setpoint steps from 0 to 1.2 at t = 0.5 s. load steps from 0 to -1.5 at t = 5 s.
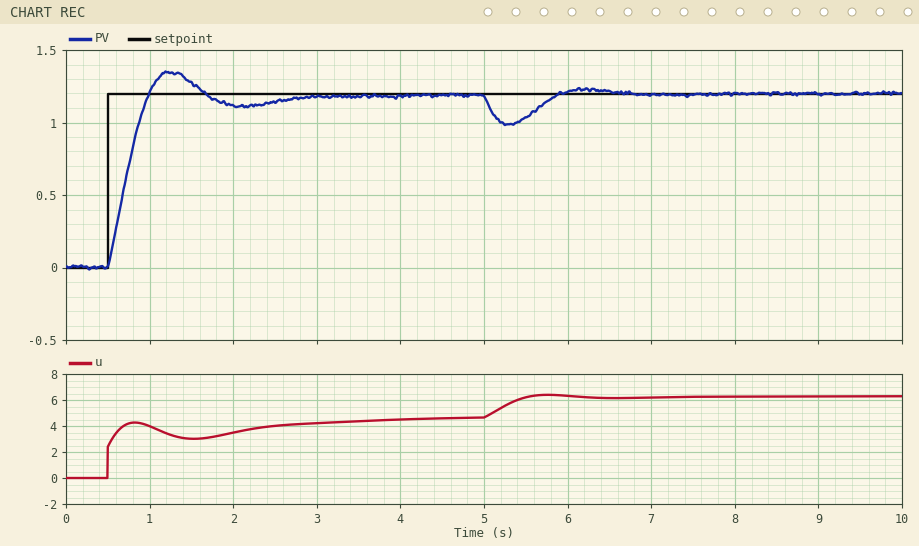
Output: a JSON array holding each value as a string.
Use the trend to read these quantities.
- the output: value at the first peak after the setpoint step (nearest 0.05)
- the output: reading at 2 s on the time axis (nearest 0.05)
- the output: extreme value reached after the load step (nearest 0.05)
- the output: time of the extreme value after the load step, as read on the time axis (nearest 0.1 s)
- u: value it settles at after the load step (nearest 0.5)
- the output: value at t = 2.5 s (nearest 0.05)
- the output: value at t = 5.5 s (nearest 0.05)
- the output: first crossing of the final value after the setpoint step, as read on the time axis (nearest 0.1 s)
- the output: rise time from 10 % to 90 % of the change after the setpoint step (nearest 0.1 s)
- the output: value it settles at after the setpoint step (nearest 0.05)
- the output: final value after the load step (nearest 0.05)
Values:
["1.35", "1.10", "1.00", "5.3 s", "6.5", "1.15", "1.05", "1.0 s", "0.4 s", "1.20", "1.20"]
